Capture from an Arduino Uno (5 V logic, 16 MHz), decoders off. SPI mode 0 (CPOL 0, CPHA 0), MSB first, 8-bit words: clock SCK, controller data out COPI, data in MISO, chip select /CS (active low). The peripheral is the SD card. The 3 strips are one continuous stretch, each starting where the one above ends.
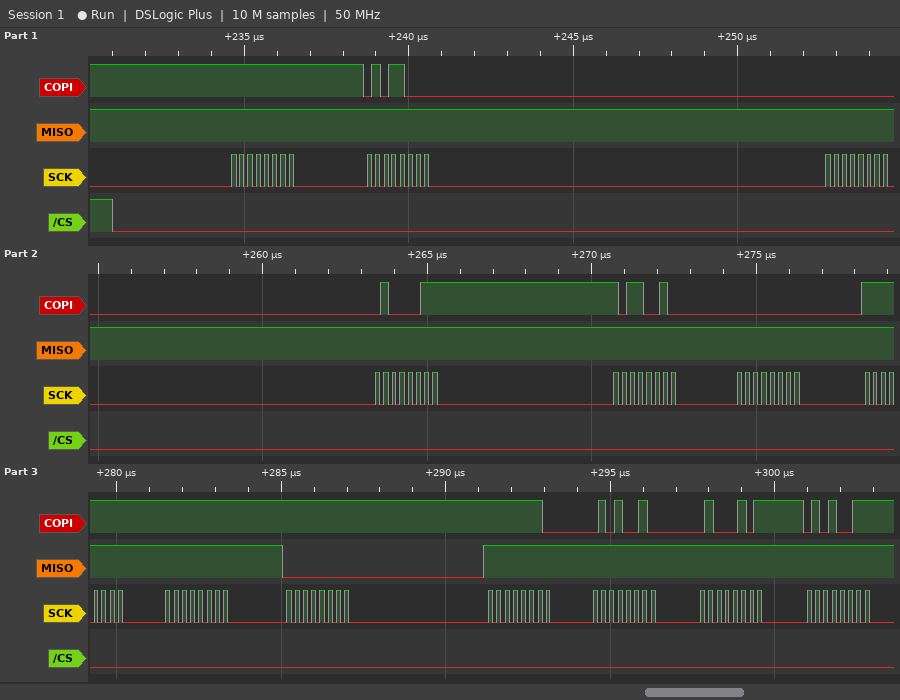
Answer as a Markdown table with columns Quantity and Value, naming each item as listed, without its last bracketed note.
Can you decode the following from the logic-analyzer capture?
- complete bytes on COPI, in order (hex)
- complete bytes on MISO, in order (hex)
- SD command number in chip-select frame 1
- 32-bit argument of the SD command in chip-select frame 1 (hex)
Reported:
| Quantity | Value |
|---|---|
| complete bytes on COPI, in order | FF 58 00 43 B2 00 FF FF FF FE 52 45 53 |
| complete bytes on MISO, in order | FF FF FF FF FF FF FF FF 00 FF FF FF FF |
| SD command number in chip-select frame 1 | CMD24 |
| 32-bit argument of the SD command in chip-select frame 1 | 0x0043B200 |
